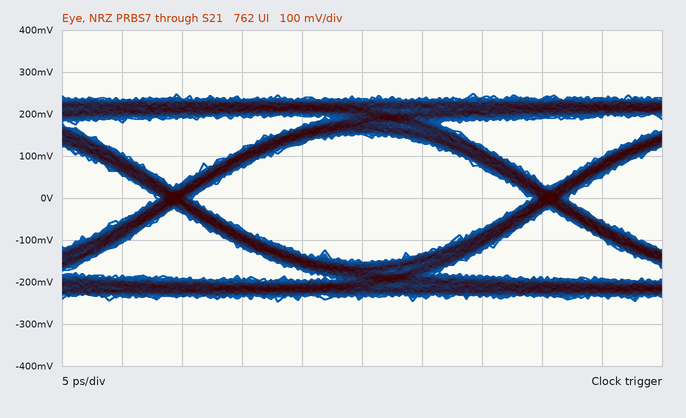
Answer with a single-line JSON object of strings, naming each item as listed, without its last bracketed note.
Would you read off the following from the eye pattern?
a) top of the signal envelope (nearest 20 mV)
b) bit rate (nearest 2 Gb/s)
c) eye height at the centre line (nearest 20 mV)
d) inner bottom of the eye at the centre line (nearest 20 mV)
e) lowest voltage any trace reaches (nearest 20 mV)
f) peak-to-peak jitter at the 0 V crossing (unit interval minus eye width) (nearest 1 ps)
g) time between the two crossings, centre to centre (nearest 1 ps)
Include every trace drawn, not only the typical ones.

{"top of the signal envelope": "240 mV", "bit rate": "32 Gb/s", "eye height at the centre line": "300 mV", "inner bottom of the eye at the centre line": "-160 mV", "lowest voltage any trace reaches": "-240 mV", "peak-to-peak jitter at the 0 V crossing (unit interval minus eye width)": "3 ps", "time between the two crossings, centre to centre": "31 ps"}
